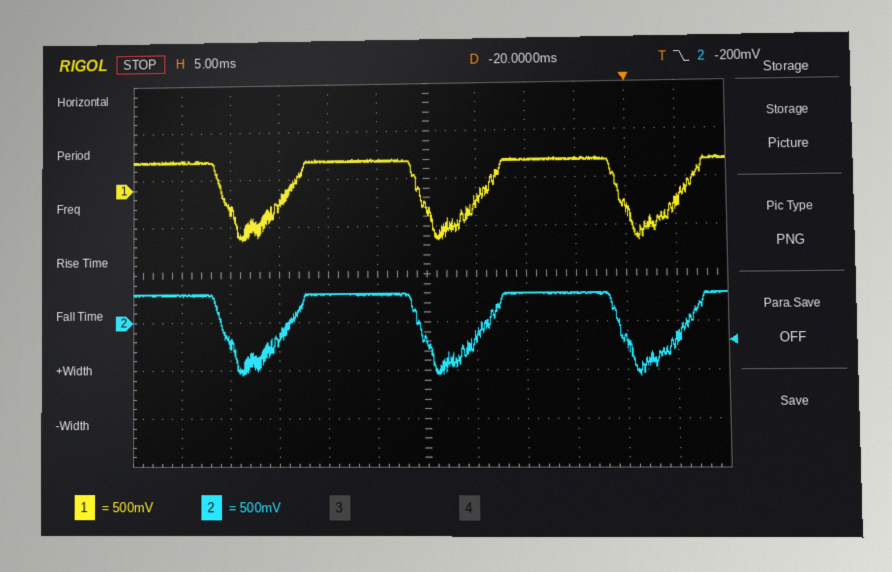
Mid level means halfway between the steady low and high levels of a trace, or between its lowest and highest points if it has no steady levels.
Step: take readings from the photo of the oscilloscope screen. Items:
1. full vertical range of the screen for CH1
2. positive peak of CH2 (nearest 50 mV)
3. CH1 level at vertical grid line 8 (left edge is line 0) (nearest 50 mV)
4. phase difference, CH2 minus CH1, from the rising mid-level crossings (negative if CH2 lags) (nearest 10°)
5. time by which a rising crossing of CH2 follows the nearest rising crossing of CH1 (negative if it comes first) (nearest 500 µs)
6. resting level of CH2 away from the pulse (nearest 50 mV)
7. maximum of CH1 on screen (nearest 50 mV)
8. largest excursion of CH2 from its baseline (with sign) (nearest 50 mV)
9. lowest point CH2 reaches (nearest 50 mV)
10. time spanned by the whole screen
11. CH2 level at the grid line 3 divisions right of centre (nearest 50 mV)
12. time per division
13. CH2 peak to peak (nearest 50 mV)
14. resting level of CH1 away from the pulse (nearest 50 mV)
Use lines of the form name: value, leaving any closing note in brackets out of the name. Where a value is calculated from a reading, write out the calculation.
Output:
full vertical range of the screen for CH1: 4 V
positive peak of CH2: 300 mV
CH1 level at vertical grid line 8 (left edge is line 0): 300 mV
phase difference, CH2 minus CH1, from the rising mid-level crossings (negative if CH2 lags): 0°
time by which a rising crossing of CH2 follows the nearest rising crossing of CH1 (negative if it comes first): 0.0 ms
resting level of CH2 away from the pulse: 300 mV
maximum of CH1 on screen: 300 mV
largest excursion of CH2 from its baseline (with sign): -550 mV − (300 mV) = -850 mV
lowest point CH2 reaches: -550 mV
time spanned by the whole screen: 60 ms
CH2 level at the grid line 3 divisions right of centre: 300 mV
time per division: 5 ms
CH2 peak to peak: 300 mV − (-550 mV) = 850 mV
resting level of CH1 away from the pulse: 300 mV
